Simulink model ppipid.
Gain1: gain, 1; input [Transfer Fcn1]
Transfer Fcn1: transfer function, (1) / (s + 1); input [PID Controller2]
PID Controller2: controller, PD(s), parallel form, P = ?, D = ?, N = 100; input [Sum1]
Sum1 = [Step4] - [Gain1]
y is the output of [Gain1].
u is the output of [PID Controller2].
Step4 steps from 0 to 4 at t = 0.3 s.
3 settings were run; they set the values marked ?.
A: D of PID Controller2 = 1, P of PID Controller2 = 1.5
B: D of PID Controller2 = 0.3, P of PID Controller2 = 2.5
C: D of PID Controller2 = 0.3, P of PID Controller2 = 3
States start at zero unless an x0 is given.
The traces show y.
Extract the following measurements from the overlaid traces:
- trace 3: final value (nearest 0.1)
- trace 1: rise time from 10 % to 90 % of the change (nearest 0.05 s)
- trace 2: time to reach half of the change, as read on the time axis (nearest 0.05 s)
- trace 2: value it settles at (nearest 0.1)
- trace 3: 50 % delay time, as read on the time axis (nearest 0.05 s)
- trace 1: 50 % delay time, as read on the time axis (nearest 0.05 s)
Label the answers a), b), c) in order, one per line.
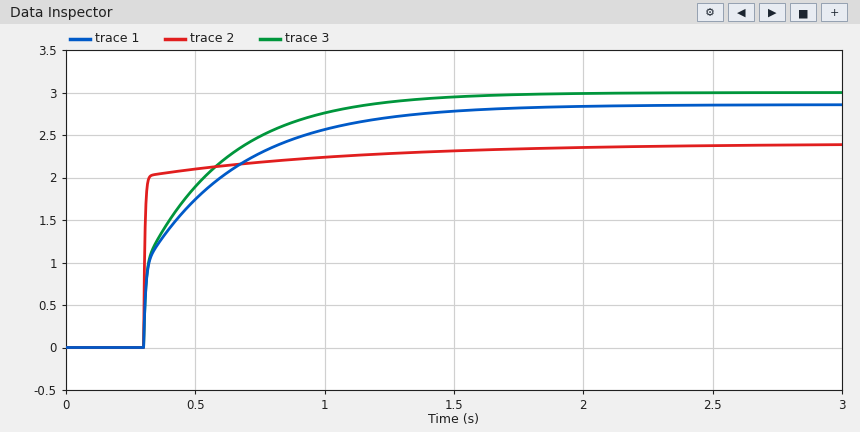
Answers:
a) 3.0
b) 0.70 s
c) 0.30 s
d) 2.4
e) 0.40 s
f) 0.40 s
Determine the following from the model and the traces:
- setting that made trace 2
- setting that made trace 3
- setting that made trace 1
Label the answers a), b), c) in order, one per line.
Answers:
a) A
b) C
c) B
